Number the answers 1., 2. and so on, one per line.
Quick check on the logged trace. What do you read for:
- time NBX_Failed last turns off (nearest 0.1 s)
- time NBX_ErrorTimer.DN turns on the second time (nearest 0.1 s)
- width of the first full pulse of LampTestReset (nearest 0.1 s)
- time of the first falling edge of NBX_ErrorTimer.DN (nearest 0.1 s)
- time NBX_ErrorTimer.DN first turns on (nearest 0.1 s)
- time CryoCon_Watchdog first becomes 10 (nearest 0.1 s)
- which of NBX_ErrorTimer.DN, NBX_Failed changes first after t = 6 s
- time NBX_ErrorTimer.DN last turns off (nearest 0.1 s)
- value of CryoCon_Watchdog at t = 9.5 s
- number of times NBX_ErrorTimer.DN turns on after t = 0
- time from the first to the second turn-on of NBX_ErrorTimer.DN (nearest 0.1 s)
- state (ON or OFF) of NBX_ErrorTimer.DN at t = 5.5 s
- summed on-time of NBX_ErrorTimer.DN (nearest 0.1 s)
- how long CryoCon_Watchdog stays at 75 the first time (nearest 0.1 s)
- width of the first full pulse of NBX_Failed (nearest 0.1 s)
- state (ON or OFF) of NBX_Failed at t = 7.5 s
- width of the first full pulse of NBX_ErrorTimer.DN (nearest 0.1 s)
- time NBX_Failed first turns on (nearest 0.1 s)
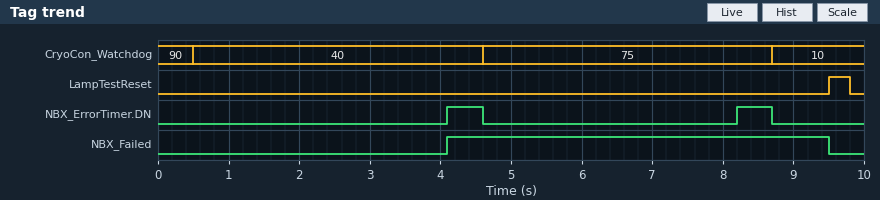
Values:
1. 9.5 s
2. 8.2 s
3. 0.3 s
4. 4.6 s
5. 4.1 s
6. 8.7 s
7. NBX_ErrorTimer.DN
8. 8.7 s
9. 10
10. 2
11. 4.1 s
12. OFF
13. 1.0 s
14. 4.1 s
15. 5.4 s
16. ON
17. 0.5 s
18. 4.1 s
